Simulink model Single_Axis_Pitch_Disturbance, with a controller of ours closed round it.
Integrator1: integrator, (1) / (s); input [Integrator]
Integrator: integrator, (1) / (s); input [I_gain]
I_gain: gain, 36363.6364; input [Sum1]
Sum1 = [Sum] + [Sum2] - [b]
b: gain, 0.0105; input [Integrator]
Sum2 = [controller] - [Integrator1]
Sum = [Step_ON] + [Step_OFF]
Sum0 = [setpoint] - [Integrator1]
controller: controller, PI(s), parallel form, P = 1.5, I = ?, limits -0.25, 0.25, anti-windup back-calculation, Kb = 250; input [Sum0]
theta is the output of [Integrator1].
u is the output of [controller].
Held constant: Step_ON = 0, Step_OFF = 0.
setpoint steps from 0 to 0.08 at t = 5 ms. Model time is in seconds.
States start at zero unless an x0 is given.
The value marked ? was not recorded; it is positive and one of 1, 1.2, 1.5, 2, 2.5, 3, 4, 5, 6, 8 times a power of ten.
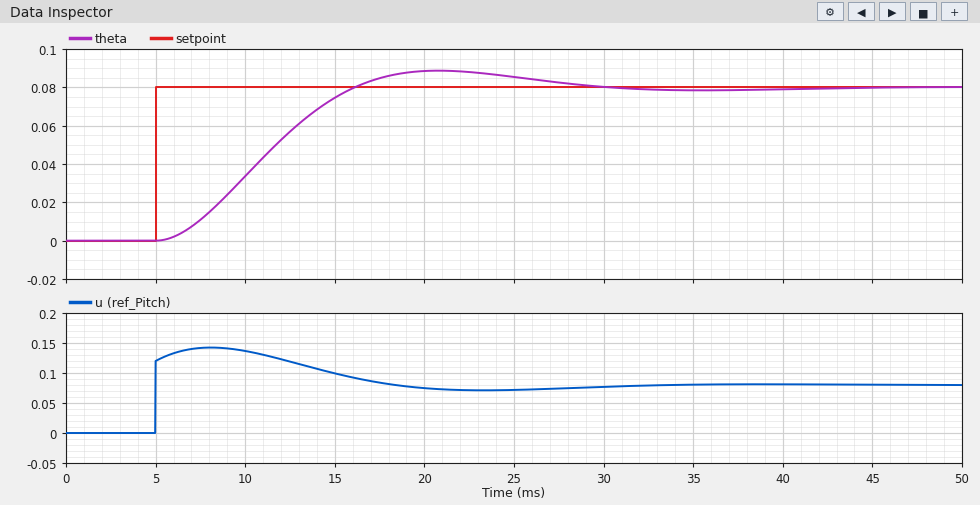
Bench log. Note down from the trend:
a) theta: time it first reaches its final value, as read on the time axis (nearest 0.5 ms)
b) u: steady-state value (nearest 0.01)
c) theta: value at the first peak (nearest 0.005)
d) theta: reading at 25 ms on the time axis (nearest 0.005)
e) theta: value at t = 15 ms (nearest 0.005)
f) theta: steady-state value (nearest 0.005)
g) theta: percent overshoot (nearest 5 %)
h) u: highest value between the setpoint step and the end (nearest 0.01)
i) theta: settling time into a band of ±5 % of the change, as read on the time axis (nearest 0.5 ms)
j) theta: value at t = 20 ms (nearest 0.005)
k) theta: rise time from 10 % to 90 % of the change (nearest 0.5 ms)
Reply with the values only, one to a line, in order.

16.0 ms
0.08
0.090
0.085
0.075
0.080
10 %
0.14
26.0 ms
0.090
7.5 ms
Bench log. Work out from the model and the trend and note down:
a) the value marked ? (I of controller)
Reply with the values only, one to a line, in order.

200
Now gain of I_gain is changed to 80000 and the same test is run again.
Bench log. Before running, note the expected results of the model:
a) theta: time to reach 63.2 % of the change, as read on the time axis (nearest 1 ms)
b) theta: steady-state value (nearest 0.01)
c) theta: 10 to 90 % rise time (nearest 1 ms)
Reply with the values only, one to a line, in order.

11 ms
0.08
9 ms
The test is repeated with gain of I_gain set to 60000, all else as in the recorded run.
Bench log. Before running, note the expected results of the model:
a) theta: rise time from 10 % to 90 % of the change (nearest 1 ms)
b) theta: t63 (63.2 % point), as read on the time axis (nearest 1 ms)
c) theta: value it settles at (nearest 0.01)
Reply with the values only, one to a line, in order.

8 ms
11 ms
0.08
